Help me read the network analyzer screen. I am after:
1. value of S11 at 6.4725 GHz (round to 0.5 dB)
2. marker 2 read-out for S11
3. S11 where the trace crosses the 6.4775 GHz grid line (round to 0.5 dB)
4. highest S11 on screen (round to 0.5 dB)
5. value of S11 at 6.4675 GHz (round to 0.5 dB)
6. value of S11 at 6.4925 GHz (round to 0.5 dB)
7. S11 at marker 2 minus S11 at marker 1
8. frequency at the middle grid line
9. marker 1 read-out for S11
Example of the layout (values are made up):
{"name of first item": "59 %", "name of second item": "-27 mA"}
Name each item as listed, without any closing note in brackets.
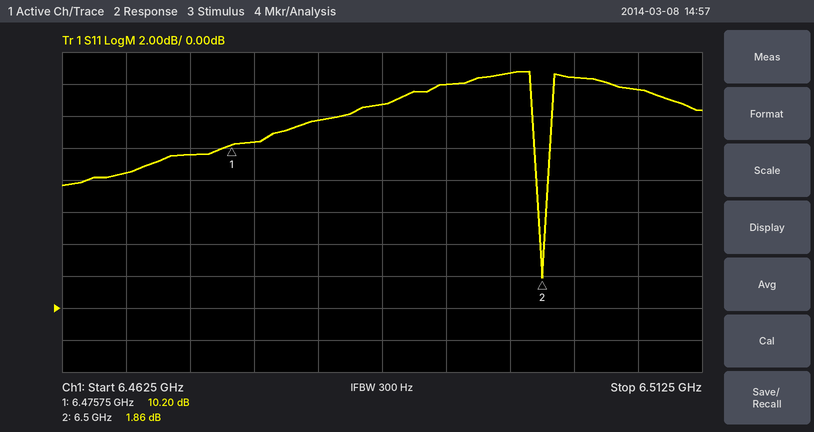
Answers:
{"value of S11 at 6.4725 GHz": "9.5 dB", "marker 2 read-out for S11": "1.86 dB", "S11 where the trace crosses the 6.4775 GHz grid line": "10.5 dB", "highest S11 on screen": "15.0 dB", "value of S11 at 6.4675 GHz": "8.5 dB", "value of S11 at 6.4925 GHz": "14.0 dB", "S11 at marker 2 minus S11 at marker 1": "-8.34 dB", "frequency at the middle grid line": "6.4875 GHz", "marker 1 read-out for S11": "10.20 dB"}
